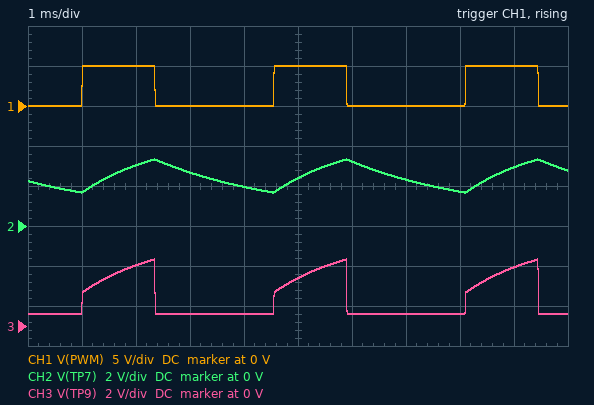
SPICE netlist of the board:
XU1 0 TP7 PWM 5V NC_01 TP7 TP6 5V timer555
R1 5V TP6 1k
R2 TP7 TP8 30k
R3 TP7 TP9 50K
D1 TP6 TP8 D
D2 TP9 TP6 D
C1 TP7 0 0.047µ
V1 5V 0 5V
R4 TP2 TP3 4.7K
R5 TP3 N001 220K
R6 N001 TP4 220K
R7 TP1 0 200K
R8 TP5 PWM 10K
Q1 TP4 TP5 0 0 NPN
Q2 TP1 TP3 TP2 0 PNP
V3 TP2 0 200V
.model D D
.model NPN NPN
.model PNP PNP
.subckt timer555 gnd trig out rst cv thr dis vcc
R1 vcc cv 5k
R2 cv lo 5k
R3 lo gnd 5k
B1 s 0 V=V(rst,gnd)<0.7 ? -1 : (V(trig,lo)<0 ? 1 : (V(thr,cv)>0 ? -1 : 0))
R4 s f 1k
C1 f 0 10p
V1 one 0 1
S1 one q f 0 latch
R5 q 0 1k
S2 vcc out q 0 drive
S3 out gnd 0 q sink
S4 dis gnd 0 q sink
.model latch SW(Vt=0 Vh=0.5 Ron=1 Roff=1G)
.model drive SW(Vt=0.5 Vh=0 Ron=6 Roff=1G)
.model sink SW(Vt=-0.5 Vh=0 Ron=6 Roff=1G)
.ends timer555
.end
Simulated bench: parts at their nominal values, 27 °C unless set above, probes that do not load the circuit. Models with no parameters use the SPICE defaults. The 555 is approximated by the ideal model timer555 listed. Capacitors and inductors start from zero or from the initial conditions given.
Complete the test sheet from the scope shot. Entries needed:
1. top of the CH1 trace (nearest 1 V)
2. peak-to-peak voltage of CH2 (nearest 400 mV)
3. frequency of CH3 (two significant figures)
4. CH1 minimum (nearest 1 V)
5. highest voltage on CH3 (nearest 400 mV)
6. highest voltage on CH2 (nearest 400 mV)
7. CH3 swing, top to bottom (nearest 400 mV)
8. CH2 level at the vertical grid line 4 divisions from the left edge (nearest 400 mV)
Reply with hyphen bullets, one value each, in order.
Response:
- 5 V
- 1.6 V
- 280 Hz
- 0 V
- 3.2 V
- 3.2 V
- 2.8 V
- 2.0 V
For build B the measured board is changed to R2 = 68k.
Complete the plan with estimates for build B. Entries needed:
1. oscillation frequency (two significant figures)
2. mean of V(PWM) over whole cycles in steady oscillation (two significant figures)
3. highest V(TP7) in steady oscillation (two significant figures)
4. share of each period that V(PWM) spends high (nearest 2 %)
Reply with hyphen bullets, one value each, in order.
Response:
- 190 Hz
- 2.9 V
- 3.3 V
- 58 %
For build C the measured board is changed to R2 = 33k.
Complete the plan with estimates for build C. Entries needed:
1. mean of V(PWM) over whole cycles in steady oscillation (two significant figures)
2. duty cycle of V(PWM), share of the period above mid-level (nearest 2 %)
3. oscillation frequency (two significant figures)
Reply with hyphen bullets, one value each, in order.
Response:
- 2.0 V
- 40 %
- 270 Hz
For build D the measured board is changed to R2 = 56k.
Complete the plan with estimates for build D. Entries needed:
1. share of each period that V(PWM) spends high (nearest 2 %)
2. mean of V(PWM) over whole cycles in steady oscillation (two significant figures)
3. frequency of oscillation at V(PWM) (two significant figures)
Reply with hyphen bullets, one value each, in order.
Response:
- 52 %
- 2.6 V
- 210 Hz
